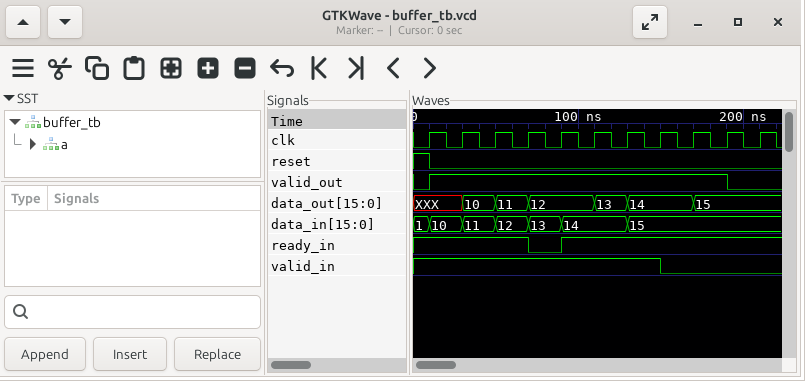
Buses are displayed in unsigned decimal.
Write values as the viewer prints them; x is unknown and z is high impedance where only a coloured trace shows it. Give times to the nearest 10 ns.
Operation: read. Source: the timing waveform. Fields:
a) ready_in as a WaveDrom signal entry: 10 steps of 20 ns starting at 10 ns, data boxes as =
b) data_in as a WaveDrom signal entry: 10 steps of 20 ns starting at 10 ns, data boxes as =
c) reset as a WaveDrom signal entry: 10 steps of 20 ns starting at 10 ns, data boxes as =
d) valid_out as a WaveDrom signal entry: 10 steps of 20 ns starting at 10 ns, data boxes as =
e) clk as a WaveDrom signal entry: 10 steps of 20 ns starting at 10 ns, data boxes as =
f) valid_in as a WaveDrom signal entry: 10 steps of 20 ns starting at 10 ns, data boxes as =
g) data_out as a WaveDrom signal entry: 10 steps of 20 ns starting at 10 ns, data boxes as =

{name: 'ready_in', wave: '1..01.....'}
{name: 'data_in', wave: '=====.=...', data: '10 11 12 13 14 15'}
{name: 'reset', wave: '0.........'}
{name: 'valid_out', wave: '1........0'}
{name: 'clk', wave: 'p.........'}
{name: 'valid_in', wave: '1......0..'}
{name: 'data_out', wave: 'x===.==.=.', data: '10 11 12 13 14 15'}
